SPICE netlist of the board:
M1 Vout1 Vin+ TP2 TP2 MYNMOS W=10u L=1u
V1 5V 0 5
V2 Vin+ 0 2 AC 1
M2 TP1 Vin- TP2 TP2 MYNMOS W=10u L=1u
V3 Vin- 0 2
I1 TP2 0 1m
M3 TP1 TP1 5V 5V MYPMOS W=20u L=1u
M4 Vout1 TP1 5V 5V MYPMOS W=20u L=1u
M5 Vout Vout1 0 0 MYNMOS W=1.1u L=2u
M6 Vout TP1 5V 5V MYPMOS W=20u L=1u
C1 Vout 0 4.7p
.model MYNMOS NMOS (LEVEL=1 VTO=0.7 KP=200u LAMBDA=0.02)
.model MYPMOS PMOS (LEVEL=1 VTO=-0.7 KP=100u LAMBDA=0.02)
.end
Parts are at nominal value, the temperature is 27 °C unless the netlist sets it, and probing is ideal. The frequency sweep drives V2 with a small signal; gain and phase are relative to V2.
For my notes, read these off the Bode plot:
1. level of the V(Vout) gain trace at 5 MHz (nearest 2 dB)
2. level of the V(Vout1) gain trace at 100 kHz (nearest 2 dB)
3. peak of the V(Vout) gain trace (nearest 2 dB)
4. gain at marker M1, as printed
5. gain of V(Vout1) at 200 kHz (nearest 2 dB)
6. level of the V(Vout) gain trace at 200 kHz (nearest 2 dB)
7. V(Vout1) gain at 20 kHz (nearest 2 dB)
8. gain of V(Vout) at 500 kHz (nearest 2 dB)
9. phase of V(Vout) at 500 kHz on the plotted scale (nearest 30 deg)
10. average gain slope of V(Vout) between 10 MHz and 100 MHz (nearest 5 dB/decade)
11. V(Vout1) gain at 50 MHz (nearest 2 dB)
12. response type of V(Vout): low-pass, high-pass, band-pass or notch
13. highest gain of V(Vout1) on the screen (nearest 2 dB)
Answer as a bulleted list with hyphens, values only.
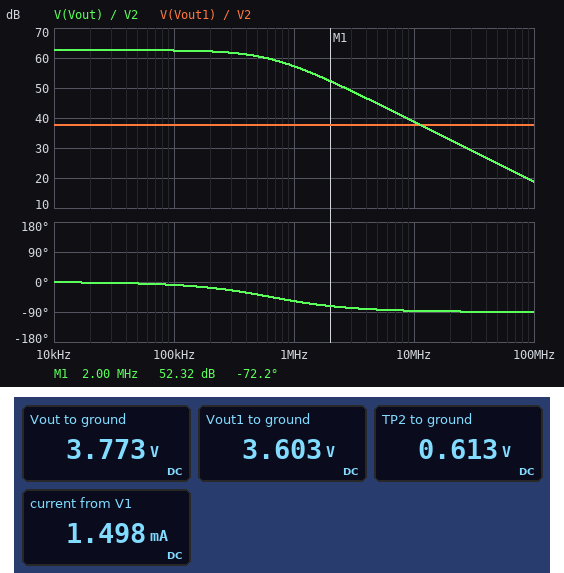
- 44 dB
- 38 dB
- 62 dB
- 52.32 dB
- 38 dB
- 62 dB
- 38 dB
- 60 dB
- -30 deg
- -20 dB/decade
- 38 dB
- low-pass
- 38 dB
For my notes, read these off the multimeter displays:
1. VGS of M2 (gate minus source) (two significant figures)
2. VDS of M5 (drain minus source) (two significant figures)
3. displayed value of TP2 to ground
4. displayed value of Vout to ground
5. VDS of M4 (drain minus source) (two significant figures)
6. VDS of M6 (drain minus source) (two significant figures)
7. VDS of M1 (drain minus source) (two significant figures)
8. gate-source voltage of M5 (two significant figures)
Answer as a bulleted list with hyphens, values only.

- 1.4 V
- 3.8 V
- 0.613 V
- 3.773 V
- -1.4 V
- -1.2 V
- 3.0 V
- 3.6 V
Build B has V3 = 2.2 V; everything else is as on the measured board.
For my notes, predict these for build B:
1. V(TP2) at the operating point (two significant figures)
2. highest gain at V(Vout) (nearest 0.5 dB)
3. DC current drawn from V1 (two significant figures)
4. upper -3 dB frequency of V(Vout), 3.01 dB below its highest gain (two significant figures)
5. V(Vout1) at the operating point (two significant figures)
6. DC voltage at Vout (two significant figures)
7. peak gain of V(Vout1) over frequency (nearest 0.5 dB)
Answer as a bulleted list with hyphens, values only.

- 720 mV
- 6.0 dB
- 1.7 mA
- 9.2 MHz
- 4.7 V
- 1.9 V
- -1.0 dB
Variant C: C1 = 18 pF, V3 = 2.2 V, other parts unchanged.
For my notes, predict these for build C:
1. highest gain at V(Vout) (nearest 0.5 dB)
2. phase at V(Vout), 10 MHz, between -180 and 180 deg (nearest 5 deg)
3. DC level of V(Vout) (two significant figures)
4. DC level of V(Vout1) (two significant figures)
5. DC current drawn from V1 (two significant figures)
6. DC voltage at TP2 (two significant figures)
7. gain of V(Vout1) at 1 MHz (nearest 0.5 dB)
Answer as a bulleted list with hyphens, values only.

- 6.0 dB
- 105 deg
- 1.9 V
- 4.7 V
- 1.7 mA
- 720 mV
- -1.0 dB
